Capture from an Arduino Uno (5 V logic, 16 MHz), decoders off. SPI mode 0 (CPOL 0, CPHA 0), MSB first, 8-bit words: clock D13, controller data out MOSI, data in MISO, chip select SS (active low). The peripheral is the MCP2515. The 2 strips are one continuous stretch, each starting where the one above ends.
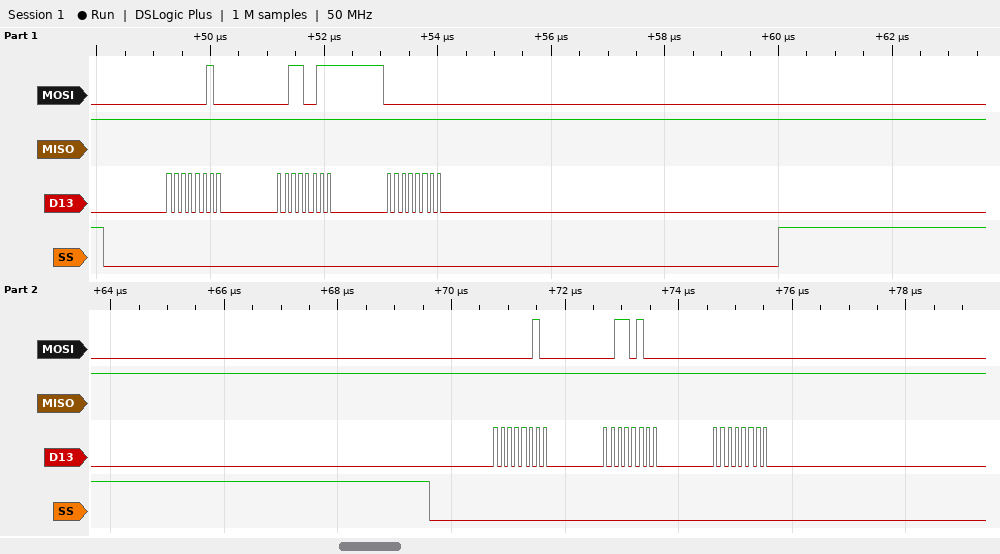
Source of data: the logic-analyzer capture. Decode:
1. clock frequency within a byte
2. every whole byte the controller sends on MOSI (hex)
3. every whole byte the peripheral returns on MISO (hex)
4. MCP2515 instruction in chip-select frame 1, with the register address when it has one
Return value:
8 MHz
0x02 0x33 0x00 0x02 0x34 0x00
0xFF 0xFF 0xFF 0xFF 0xFF 0xFF
WRITE 0x33
